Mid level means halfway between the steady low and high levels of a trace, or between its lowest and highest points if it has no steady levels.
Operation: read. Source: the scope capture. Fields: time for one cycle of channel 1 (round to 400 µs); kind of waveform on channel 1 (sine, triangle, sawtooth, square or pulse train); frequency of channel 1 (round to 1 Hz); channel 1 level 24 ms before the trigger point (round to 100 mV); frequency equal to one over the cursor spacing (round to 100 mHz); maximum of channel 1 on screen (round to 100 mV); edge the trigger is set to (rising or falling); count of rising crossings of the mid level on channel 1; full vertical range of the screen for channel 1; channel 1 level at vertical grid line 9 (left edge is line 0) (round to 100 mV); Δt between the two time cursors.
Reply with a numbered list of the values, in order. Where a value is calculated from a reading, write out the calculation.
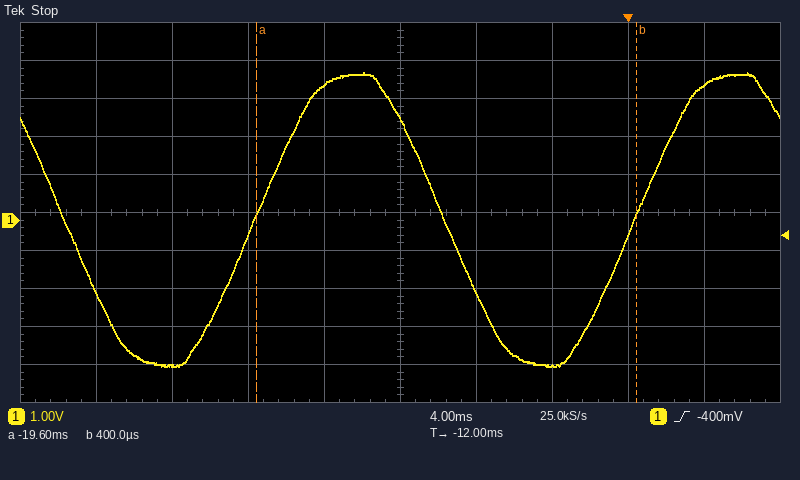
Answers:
1. 20.0 ms
2. sine
3. 1 / 20.0 ms ≈ 50 Hz
4. -3.8 V
5. 1 / 20.0 ms ≈ 50.0 Hz
6. 3.9 V
7. rising
8. 2
9. 10 V
10. 3.6 V
11. 400 µs − (-19.6 ms) = 20.0 ms
